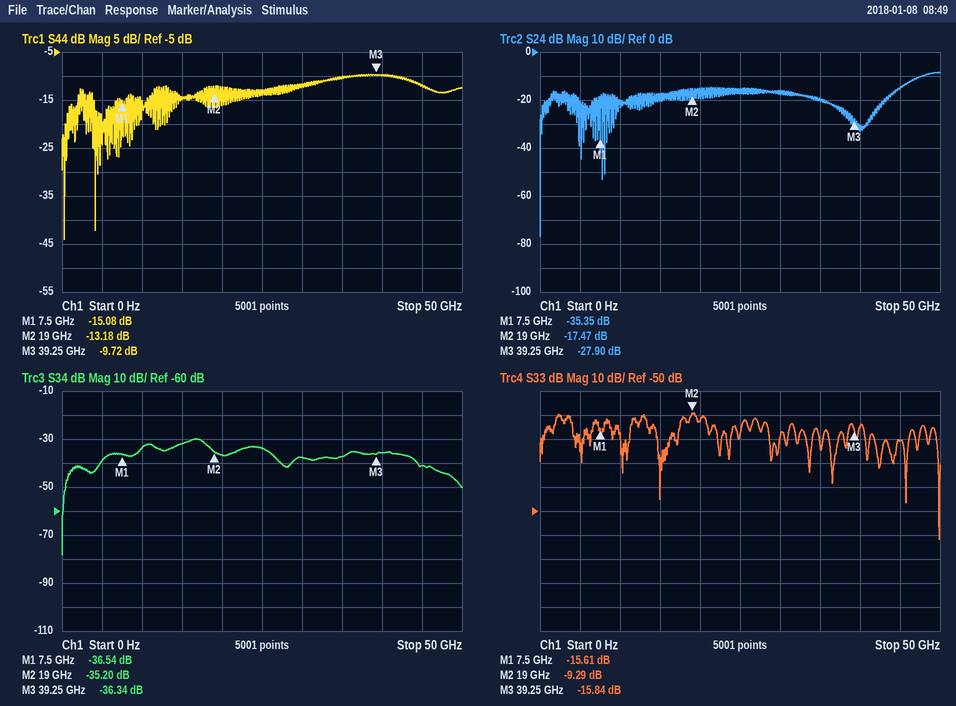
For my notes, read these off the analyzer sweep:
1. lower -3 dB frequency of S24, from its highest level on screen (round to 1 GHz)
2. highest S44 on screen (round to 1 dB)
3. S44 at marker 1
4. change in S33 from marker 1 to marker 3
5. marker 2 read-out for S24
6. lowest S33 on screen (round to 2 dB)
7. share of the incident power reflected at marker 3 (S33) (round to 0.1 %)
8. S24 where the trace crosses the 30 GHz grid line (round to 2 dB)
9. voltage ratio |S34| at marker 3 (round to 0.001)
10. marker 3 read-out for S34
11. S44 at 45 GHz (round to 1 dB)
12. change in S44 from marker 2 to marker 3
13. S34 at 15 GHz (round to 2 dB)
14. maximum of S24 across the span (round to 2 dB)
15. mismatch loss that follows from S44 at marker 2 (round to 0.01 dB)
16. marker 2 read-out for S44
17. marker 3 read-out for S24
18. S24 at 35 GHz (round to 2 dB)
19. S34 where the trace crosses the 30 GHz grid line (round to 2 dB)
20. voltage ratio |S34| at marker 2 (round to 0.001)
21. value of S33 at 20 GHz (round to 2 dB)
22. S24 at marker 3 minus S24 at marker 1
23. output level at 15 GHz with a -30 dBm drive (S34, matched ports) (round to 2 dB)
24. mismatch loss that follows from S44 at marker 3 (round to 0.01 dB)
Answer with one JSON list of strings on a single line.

["47 GHz", "-10 dB", "-15.08 dB", "-0.23 dB", "-17.47 dB", "-62 dB", "2.6 %", "-16 dB", "0.015", "-36.34 dB", "-12 dB", "3.46 dB", "-32 dB", "-8 dB", "0.21 dB", "-13.18 dB", "-27.90 dB", "-20 dB", "-38 dB", "0.017", "-12 dB", "7.45 dB", "-62 dBm", "0.49 dB"]
